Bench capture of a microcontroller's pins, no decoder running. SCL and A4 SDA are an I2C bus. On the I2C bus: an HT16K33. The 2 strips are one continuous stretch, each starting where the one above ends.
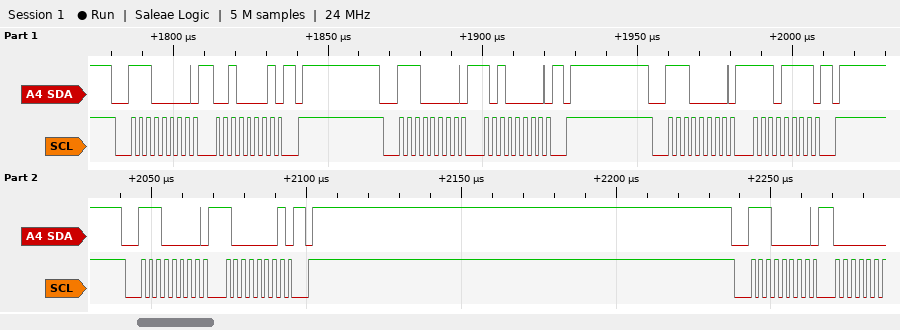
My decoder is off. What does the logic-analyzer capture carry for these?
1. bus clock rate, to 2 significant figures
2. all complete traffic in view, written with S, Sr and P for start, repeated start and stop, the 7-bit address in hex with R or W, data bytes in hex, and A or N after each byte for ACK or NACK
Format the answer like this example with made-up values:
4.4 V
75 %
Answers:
400 kHz
S 70W A 21 A P S 70W A A0 A P S 70W A EF A P S 70W A 81 A P S 70W A
